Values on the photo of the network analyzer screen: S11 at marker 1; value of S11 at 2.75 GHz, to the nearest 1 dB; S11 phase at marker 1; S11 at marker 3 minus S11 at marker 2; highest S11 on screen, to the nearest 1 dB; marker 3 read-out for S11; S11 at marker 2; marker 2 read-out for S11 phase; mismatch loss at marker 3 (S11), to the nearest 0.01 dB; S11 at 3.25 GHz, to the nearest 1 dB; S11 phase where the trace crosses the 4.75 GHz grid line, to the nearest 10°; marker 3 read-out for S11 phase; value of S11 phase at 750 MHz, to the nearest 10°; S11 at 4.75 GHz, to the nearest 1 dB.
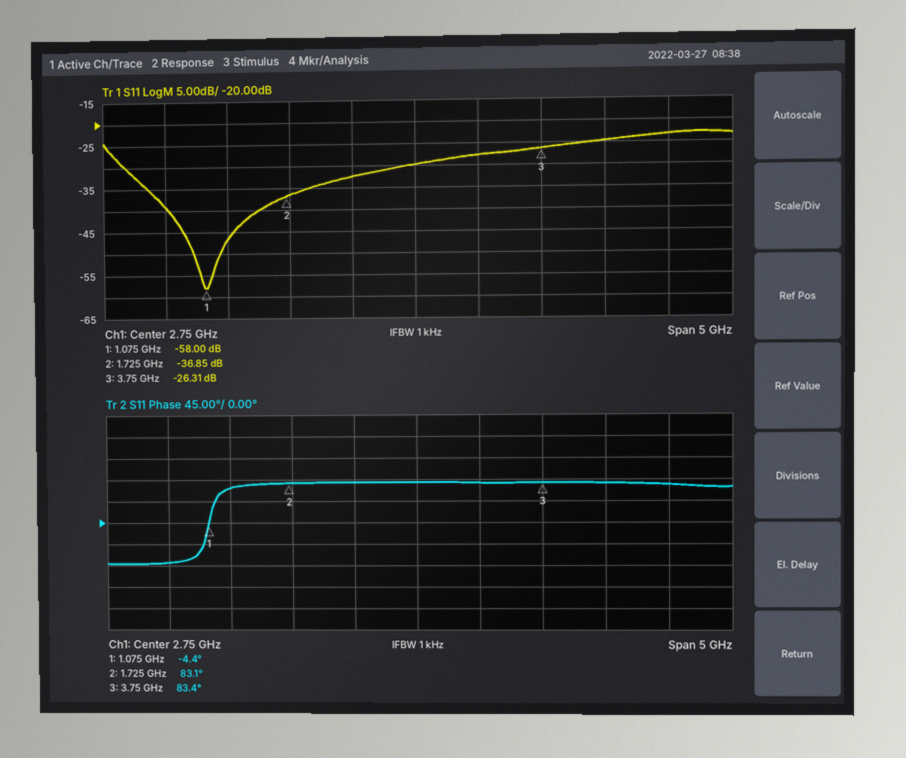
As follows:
-58.00 dB
-30 dB
-4.4°
10.54 dB
-23 dB
-26.31 dB
-36.85 dB
83.1°
0.01 dB
-28 dB
80°
83.4°
-80°
-23 dB
